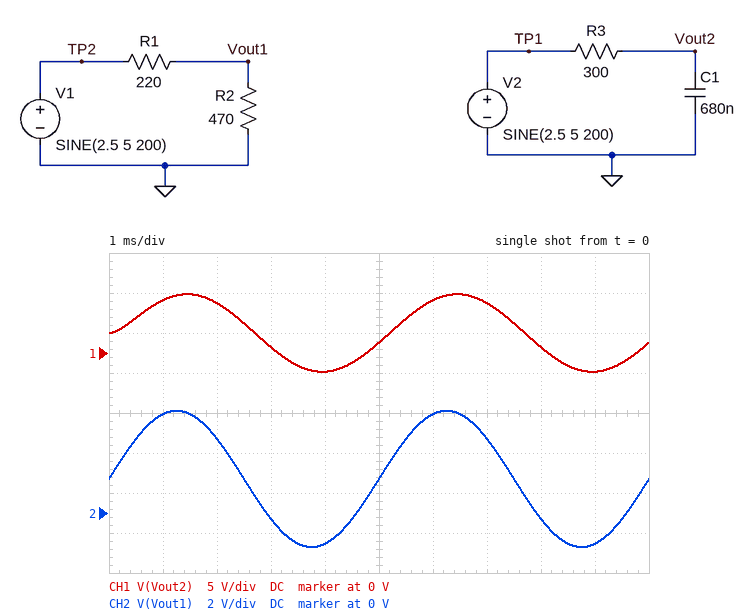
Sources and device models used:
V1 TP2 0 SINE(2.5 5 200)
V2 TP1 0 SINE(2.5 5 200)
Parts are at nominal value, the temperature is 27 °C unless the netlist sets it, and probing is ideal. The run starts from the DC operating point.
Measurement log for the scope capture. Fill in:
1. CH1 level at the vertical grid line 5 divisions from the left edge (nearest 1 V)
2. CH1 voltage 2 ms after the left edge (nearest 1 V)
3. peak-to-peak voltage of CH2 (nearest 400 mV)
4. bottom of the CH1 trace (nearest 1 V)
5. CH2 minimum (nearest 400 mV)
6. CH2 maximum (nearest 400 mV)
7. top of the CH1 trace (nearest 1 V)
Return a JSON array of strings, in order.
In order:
["1 V", "6 V", "6.8 V", "-2 V", "-1.6 V", "5.2 V", "7 V"]
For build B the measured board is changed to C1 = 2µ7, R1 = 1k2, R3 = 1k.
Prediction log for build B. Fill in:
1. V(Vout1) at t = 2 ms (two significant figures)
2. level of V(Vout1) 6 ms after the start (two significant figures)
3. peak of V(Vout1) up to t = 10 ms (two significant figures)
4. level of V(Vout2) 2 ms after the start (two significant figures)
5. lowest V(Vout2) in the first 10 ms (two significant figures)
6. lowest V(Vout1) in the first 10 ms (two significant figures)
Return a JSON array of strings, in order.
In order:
["1.5 V", "2.0 V", "2.1 V", "4.5 V", "1.1 V", "-700 mV"]
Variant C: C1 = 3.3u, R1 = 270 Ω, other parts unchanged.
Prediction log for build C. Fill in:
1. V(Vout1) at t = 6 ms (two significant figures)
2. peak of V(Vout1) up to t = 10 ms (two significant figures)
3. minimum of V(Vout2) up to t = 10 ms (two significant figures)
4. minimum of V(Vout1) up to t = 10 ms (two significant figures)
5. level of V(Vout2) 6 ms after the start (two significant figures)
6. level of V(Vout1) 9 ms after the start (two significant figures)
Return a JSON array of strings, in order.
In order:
["4.6 V", "4.8 V", "-630 mV", "-1.6 V", "3.6 V", "-1.4 V"]
